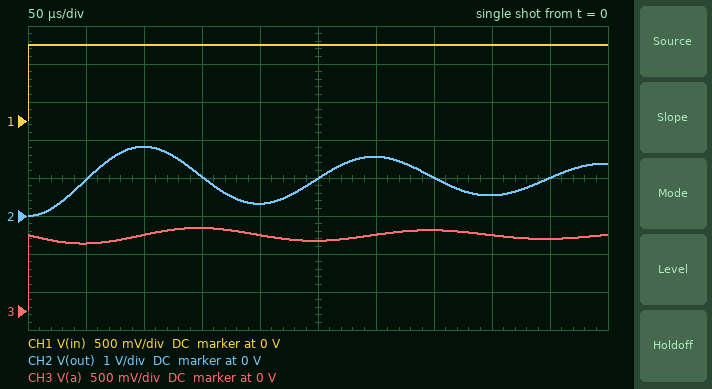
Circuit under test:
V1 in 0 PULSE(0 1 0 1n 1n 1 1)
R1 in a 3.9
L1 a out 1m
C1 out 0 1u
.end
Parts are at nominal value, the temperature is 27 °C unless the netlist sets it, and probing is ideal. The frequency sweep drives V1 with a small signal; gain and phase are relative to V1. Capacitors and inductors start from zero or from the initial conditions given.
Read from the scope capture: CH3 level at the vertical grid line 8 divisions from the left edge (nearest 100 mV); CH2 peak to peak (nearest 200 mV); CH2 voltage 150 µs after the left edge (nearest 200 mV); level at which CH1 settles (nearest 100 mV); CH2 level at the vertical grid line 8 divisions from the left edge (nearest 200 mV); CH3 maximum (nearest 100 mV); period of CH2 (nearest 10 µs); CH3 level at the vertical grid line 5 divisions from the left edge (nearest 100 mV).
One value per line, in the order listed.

1.0 V
1.8 V
1.0 V
1.0 V
600 mV
1.1 V
200 µs
900 mV
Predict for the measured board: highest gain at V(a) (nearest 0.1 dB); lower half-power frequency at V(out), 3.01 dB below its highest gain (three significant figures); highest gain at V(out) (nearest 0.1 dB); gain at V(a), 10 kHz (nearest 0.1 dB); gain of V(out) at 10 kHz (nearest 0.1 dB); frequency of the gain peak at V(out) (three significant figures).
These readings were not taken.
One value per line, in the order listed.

0 dB
4.69 kHz
18.2 dB
0 dB
-9.4 dB
5.01 kHz
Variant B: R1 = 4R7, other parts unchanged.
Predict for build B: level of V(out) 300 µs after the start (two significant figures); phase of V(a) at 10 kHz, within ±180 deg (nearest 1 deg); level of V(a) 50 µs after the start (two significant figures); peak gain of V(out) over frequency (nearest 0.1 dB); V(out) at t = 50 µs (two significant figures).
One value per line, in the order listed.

1.5 V
6 deg
870 mV
16.6 dB
940 mV
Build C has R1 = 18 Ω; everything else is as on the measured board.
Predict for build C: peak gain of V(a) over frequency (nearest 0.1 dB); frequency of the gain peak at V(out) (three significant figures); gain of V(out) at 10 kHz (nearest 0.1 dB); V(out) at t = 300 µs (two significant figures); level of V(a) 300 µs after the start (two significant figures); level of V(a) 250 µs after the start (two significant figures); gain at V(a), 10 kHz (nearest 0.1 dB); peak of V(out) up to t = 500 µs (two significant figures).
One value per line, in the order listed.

0 dB
4.61 kHz
-10.0 dB
1.1 V
990 mV
940 mV
-0.6 dB
1.4 V
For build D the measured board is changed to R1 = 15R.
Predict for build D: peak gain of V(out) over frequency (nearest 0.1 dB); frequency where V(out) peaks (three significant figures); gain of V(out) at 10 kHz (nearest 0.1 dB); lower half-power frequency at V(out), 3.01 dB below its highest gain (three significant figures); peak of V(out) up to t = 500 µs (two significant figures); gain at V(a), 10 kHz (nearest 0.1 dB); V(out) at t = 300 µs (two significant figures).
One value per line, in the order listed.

6.7 dB
4.74 kHz
-9.8 dB
3.29 kHz
1.5 V
-0.4 dB
1.1 V
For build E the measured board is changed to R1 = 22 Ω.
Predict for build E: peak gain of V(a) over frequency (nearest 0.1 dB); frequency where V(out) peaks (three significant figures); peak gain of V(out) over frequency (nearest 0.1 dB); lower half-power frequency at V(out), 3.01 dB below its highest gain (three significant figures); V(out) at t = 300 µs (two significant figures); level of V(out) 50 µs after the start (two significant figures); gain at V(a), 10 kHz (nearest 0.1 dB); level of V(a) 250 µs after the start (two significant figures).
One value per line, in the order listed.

0 dB
4.38 kHz
3.7 dB
1.64 kHz
1.0 V
740 mV
-0.9 dB
960 mV
